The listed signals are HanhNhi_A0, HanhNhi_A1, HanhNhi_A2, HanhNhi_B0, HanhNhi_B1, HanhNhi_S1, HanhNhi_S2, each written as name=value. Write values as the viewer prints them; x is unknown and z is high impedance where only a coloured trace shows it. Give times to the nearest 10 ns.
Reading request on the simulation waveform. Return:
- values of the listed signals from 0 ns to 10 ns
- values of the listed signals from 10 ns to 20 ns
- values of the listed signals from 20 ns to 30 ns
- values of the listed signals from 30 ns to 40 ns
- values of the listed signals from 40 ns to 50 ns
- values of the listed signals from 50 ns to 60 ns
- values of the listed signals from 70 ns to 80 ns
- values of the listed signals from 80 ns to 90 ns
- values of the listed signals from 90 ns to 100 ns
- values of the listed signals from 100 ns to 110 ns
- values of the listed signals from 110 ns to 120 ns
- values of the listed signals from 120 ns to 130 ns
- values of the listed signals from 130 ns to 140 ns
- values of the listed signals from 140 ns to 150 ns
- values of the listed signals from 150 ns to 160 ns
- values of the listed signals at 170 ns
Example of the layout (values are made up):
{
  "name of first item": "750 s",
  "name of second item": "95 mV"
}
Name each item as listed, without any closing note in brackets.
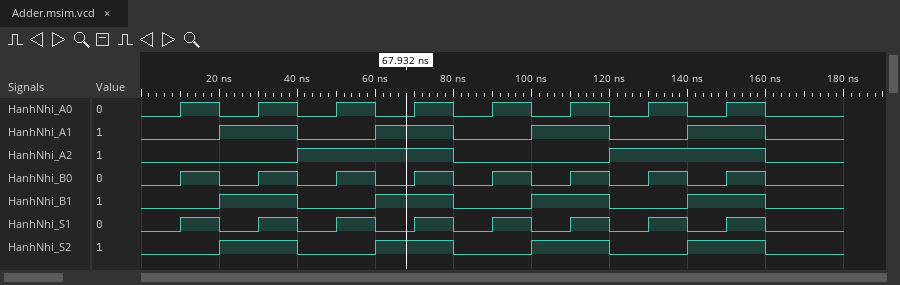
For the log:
{
  "values of the listed signals from 0 ns to 10 ns": "HanhNhi_A0=0, HanhNhi_A1=0, HanhNhi_A2=0, HanhNhi_B0=0, HanhNhi_B1=0, HanhNhi_S1=0, HanhNhi_S2=0",
  "values of the listed signals from 10 ns to 20 ns": "HanhNhi_A0=1, HanhNhi_A1=0, HanhNhi_A2=0, HanhNhi_B0=1, HanhNhi_B1=0, HanhNhi_S1=1, HanhNhi_S2=0",
  "values of the listed signals from 20 ns to 30 ns": "HanhNhi_A0=0, HanhNhi_A1=1, HanhNhi_A2=0, HanhNhi_B0=0, HanhNhi_B1=1, HanhNhi_S1=0, HanhNhi_S2=1",
  "values of the listed signals from 30 ns to 40 ns": "HanhNhi_A0=1, HanhNhi_A1=1, HanhNhi_A2=0, HanhNhi_B0=1, HanhNhi_B1=1, HanhNhi_S1=1, HanhNhi_S2=1",
  "values of the listed signals from 40 ns to 50 ns": "HanhNhi_A0=0, HanhNhi_A1=0, HanhNhi_A2=1, HanhNhi_B0=0, HanhNhi_B1=0, HanhNhi_S1=0, HanhNhi_S2=0",
  "values of the listed signals from 50 ns to 60 ns": "HanhNhi_A0=1, HanhNhi_A1=0, HanhNhi_A2=1, HanhNhi_B0=1, HanhNhi_B1=0, HanhNhi_S1=1, HanhNhi_S2=0",
  "values of the listed signals from 70 ns to 80 ns": "HanhNhi_A0=1, HanhNhi_A1=1, HanhNhi_A2=1, HanhNhi_B0=1, HanhNhi_B1=1, HanhNhi_S1=1, HanhNhi_S2=1",
  "values of the listed signals from 80 ns to 90 ns": "HanhNhi_A0=0, HanhNhi_A1=0, HanhNhi_A2=0, HanhNhi_B0=0, HanhNhi_B1=0, HanhNhi_S1=0, HanhNhi_S2=0",
  "values of the listed signals from 90 ns to 100 ns": "HanhNhi_A0=1, HanhNhi_A1=0, HanhNhi_A2=0, HanhNhi_B0=1, HanhNhi_B1=0, HanhNhi_S1=1, HanhNhi_S2=0",
  "values of the listed signals from 100 ns to 110 ns": "HanhNhi_A0=0, HanhNhi_A1=1, HanhNhi_A2=0, HanhNhi_B0=0, HanhNhi_B1=1, HanhNhi_S1=0, HanhNhi_S2=1",
  "values of the listed signals from 110 ns to 120 ns": "HanhNhi_A0=1, HanhNhi_A1=1, HanhNhi_A2=0, HanhNhi_B0=1, HanhNhi_B1=1, HanhNhi_S1=1, HanhNhi_S2=1",
  "values of the listed signals from 120 ns to 130 ns": "HanhNhi_A0=0, HanhNhi_A1=0, HanhNhi_A2=1, HanhNhi_B0=0, HanhNhi_B1=0, HanhNhi_S1=0, HanhNhi_S2=0",
  "values of the listed signals from 130 ns to 140 ns": "HanhNhi_A0=1, HanhNhi_A1=0, HanhNhi_A2=1, HanhNhi_B0=1, HanhNhi_B1=0, HanhNhi_S1=1, HanhNhi_S2=0",
  "values of the listed signals from 140 ns to 150 ns": "HanhNhi_A0=0, HanhNhi_A1=1, HanhNhi_A2=1, HanhNhi_B0=0, HanhNhi_B1=1, HanhNhi_S1=0, HanhNhi_S2=1",
  "values of the listed signals from 150 ns to 160 ns": "HanhNhi_A0=1, HanhNhi_A1=1, HanhNhi_A2=1, HanhNhi_B0=1, HanhNhi_B1=1, HanhNhi_S1=1, HanhNhi_S2=1",
  "values of the listed signals at 170 ns": "HanhNhi_A0=0, HanhNhi_A1=0, HanhNhi_A2=0, HanhNhi_B0=0, HanhNhi_B1=0, HanhNhi_S1=0, HanhNhi_S2=0"
}
